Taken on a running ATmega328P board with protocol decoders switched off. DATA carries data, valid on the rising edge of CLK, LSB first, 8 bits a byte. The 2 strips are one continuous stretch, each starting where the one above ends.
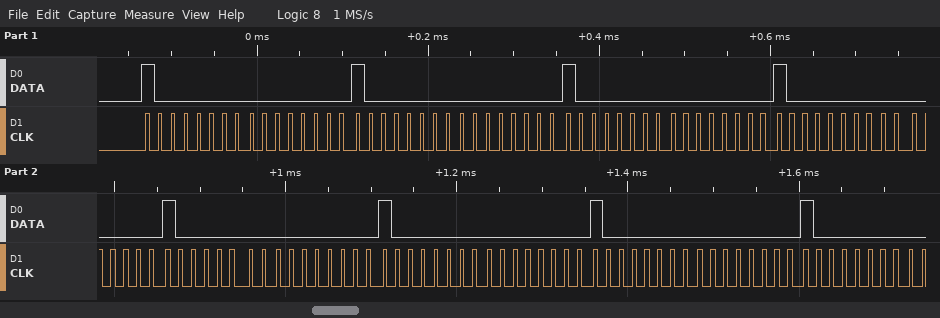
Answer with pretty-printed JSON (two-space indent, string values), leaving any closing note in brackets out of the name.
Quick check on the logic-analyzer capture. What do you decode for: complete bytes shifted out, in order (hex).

{
  "complete bytes shifted out, in order": "0x01 0x00 0x01 0x00 0x01 0x00 0x01 0x00 0x01 0x00 0x01 0x00 0x01 0x00 0x01"
}
